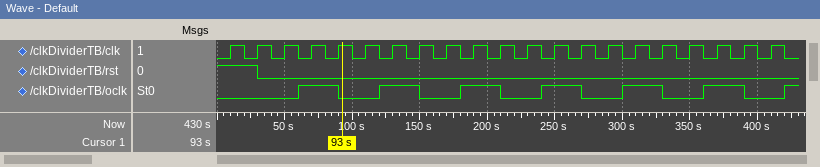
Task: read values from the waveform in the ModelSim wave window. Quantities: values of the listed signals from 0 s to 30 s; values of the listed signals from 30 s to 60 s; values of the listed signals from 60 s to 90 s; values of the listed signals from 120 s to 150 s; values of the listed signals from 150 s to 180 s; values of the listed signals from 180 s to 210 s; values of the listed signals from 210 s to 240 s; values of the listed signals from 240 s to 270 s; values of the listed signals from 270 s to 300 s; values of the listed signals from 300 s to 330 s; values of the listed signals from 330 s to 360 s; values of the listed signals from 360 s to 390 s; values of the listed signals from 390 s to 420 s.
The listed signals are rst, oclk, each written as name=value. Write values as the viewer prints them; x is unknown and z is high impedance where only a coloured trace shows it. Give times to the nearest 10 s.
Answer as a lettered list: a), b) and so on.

a) rst=1, oclk=0
b) rst=0, oclk=0
c) rst=0, oclk=1
d) rst=0, oclk=1
e) rst=0, oclk=0
f) rst=0, oclk=1
g) rst=0, oclk=0
h) rst=0, oclk=1
i) rst=0, oclk=0
j) rst=0, oclk=1
k) rst=0, oclk=0
l) rst=0, oclk=1
m) rst=0, oclk=0
